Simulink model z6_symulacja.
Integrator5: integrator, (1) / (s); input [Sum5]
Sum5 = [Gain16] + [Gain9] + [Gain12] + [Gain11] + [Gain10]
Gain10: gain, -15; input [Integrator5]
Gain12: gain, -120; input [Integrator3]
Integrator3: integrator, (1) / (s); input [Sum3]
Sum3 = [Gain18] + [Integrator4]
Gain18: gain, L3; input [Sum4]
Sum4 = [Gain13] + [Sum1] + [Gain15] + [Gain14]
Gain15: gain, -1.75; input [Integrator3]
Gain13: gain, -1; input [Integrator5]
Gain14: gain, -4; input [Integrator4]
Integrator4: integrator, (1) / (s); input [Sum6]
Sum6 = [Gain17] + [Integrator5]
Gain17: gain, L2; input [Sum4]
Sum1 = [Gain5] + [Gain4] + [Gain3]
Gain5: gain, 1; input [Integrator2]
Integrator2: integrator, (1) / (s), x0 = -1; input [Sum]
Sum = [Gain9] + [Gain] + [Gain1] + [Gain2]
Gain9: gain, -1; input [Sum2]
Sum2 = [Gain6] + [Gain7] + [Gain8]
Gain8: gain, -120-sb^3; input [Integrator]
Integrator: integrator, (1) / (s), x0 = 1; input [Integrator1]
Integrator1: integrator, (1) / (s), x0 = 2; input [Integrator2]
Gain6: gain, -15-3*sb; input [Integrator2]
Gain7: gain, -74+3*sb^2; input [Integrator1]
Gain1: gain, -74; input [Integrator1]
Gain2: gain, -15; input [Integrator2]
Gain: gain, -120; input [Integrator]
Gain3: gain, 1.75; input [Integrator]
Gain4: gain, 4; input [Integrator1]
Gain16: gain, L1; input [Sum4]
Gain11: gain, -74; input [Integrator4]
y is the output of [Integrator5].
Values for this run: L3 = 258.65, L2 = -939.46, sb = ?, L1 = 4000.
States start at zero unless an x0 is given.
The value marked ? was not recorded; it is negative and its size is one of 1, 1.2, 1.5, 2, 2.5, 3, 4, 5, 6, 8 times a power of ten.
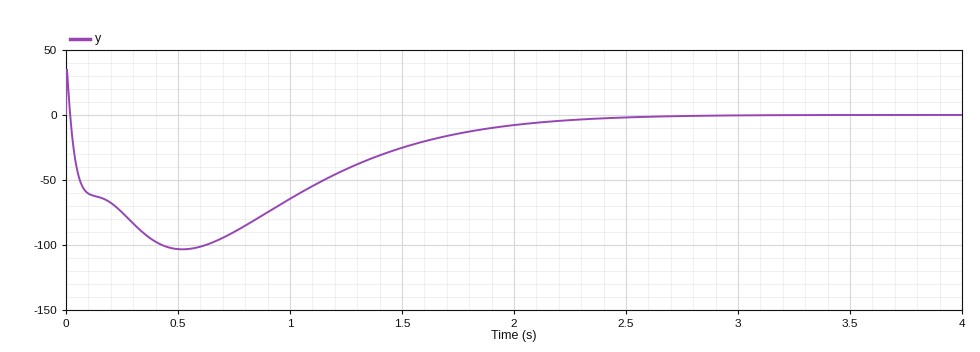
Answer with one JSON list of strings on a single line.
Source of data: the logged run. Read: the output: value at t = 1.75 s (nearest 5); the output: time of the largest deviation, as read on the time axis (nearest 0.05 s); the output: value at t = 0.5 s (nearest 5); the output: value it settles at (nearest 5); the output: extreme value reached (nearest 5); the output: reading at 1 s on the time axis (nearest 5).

["-15", "0.50 s", "-105", "0", "-105", "-65"]
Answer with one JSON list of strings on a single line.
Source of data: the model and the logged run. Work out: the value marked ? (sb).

["-12"]
